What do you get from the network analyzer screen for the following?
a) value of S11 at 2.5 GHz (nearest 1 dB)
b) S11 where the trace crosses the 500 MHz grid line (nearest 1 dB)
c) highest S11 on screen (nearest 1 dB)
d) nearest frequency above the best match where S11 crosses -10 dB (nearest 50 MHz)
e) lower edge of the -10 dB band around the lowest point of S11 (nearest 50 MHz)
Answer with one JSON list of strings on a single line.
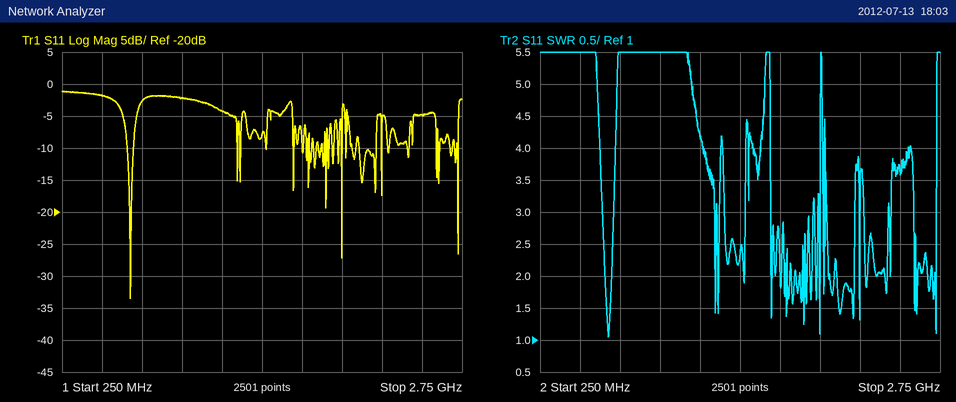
["-5 dB", "-2 dB", "-1 dB", "700 MHz", "650 MHz"]
